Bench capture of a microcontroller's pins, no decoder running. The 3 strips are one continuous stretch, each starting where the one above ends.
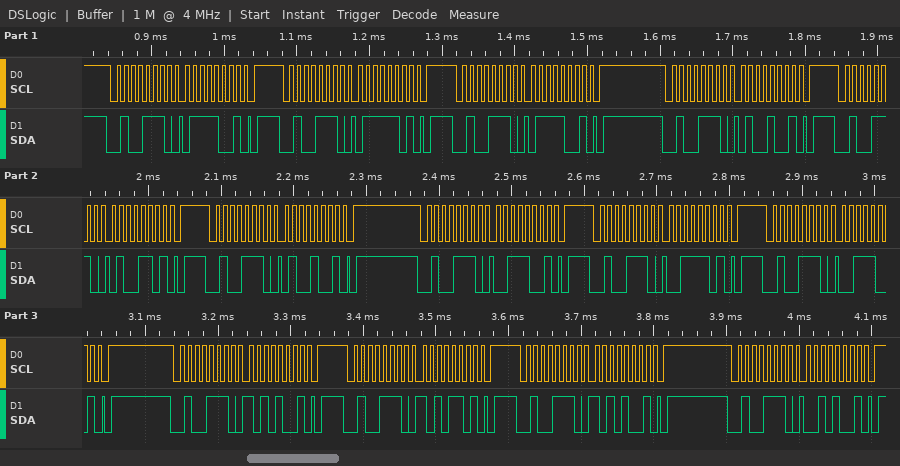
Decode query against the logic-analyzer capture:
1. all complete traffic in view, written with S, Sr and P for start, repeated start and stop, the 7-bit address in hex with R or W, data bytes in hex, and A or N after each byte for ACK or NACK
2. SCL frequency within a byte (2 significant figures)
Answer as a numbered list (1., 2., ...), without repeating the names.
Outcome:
1. S 27W A 79 A P S 27W A 7D A P S 27W A 79 A P S 27W A 49 A P S 27W A 4D A P S 27W A 49 A P S 27W A 39 A P S 27W A 3D A P S 27W A 39 A P S 27W A A9 A P S 27W A AD A P S 27W A A9 A P S 27W A 29 A P
2. 100 kHz
